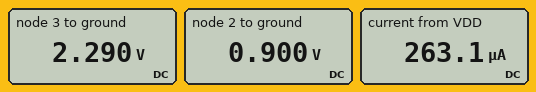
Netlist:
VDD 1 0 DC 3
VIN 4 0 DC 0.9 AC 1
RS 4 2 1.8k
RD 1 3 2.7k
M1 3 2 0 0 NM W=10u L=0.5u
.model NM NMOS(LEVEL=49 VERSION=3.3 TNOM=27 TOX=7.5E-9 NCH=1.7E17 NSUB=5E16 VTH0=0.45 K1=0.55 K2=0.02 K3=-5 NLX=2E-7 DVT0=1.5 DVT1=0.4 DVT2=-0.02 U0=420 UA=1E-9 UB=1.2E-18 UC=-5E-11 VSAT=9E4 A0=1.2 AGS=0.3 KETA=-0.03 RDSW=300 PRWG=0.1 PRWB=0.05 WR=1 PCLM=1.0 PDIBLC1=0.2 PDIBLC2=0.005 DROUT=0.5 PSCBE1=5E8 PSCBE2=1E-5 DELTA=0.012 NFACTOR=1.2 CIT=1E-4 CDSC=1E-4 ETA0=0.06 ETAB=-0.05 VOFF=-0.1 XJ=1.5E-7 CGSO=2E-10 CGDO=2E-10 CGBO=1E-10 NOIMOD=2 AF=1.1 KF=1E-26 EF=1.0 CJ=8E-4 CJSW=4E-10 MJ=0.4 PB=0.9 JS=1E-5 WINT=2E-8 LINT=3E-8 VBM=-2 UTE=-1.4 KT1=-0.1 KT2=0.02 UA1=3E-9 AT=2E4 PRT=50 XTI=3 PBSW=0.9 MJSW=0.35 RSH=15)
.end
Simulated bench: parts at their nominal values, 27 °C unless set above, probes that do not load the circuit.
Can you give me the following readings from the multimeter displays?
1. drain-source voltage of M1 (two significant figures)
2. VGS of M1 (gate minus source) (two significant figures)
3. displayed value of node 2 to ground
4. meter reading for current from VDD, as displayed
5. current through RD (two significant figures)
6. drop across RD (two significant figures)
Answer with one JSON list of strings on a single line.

["2.3 V", "900 mV", "0.900 V", "263.1 µA", "260 µA", "710 mV"]
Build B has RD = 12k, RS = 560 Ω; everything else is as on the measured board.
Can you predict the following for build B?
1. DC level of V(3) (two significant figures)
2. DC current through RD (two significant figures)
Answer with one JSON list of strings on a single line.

["440 mV", "210 µA"]
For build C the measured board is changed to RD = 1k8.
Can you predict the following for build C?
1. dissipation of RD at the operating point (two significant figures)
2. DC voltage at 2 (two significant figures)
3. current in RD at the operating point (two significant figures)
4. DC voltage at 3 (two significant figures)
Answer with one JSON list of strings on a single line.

["130 µW", "900 mV", "270 µA", "2.5 V"]
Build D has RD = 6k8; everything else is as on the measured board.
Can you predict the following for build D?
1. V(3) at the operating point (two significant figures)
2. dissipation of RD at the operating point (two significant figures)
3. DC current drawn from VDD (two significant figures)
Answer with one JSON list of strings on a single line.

["1.4 V", "400 µW", "240 µA"]
